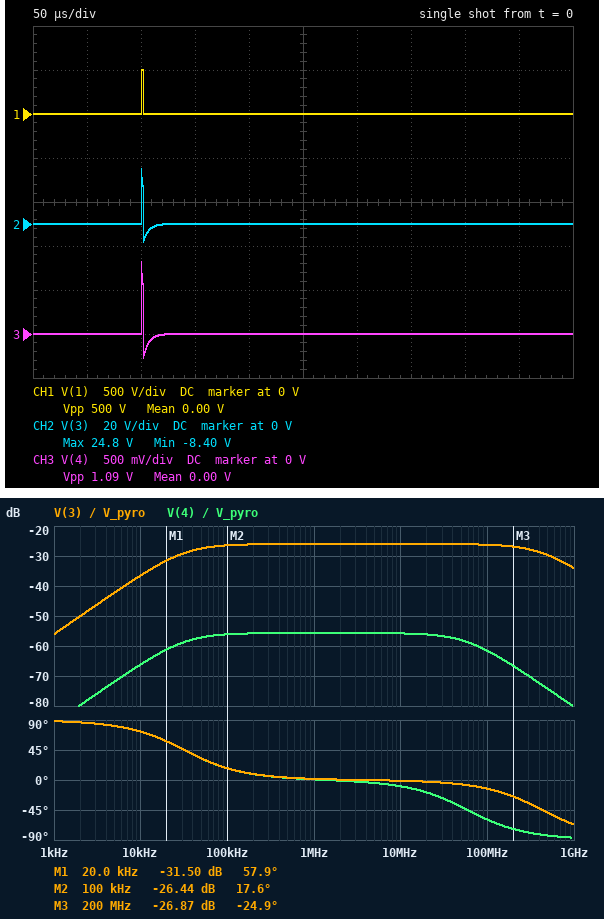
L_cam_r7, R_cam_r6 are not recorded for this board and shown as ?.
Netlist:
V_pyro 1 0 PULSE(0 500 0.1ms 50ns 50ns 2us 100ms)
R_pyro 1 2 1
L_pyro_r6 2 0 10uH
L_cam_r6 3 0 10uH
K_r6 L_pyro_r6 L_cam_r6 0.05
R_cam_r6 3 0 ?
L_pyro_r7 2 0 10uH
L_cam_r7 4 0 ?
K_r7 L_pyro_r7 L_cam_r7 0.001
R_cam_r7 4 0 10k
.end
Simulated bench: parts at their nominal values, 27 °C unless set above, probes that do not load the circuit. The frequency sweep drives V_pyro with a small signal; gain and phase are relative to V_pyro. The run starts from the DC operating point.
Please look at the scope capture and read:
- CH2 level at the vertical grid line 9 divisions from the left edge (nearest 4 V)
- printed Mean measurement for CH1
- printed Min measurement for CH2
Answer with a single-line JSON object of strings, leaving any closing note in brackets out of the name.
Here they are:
{"CH2 level at the vertical grid line 9 divisions from the left edge": "0 V", "printed Mean measurement for CH1": "0.00 V", "printed Min measurement for CH2": "-8.40 V"}
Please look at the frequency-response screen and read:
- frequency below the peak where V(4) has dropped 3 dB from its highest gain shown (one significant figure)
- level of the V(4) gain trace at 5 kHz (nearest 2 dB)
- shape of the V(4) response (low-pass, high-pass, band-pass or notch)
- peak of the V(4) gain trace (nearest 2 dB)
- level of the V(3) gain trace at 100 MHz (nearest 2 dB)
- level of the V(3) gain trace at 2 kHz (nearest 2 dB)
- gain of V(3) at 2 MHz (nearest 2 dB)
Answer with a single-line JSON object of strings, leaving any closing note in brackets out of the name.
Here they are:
{"frequency below the peak where V(4) has dropped 3 dB from its highest gain shown": "30 kHz", "level of the V(4) gain trace at 5 kHz": "-72 dB", "shape of the V(4) response": "band-pass", "peak of the V(4) gain trace": "-56 dB", "level of the V(3) gain trace at 100 MHz": "-26 dB", "level of the V(3) gain trace at 2 kHz": "-50 dB", "gain of V(3) at 2 MHz": "-26 dB"}
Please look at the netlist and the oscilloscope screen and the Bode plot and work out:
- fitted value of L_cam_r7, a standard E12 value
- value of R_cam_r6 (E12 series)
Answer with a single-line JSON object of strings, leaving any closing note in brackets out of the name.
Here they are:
{"fitted value of L_cam_r7, a standard E12 value": "27 µH", "value of R_cam_r6": "27 kΩ"}
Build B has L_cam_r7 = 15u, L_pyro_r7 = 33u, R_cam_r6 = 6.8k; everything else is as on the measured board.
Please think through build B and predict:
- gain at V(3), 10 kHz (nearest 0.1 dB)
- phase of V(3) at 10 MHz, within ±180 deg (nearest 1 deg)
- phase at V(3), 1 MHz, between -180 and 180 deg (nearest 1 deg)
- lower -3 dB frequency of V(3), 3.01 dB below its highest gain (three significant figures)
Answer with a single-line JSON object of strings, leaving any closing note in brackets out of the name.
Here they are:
{"gain at V(3), 10 kHz": "-33.3 dB", "phase of V(3) at 10 MHz, within ±180 deg": "-5 deg", "phase at V(3), 1 MHz, between -180 and 180 deg": "1 deg", "lower -3 dB frequency of V(3), 3.01 dB below its highest gain": "20.7 kHz"}
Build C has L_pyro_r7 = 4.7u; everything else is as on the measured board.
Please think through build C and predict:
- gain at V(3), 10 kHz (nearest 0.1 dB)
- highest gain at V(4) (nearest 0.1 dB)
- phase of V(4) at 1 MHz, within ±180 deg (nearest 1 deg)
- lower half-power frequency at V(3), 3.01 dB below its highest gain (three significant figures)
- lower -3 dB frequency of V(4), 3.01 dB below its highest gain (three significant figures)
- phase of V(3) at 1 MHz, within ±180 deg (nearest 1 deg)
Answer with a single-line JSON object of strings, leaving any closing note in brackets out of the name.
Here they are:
{"gain at V(3), 10 kHz": "-40.1 dB", "highest gain at V(4)": "-52.4 dB", "phase of V(4) at 1 MHz, within ±180 deg": "2 deg", "lower half-power frequency at V(3), 3.01 dB below its highest gain": "49.8 kHz", "lower -3 dB frequency of V(4), 3.01 dB below its highest gain": "49.7 kHz", "phase of V(3) at 1 MHz, within ±180 deg": "3 deg"}
